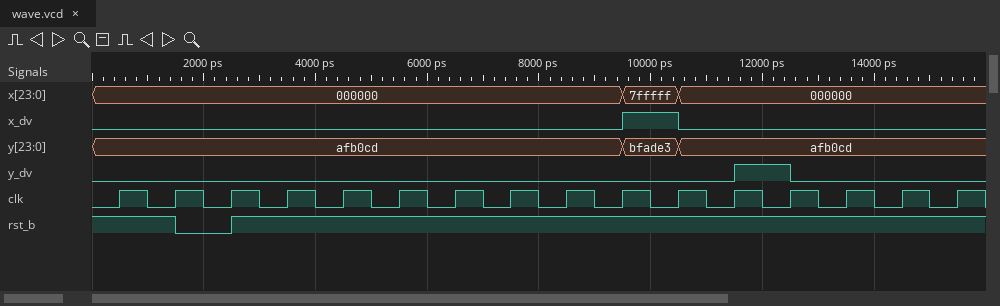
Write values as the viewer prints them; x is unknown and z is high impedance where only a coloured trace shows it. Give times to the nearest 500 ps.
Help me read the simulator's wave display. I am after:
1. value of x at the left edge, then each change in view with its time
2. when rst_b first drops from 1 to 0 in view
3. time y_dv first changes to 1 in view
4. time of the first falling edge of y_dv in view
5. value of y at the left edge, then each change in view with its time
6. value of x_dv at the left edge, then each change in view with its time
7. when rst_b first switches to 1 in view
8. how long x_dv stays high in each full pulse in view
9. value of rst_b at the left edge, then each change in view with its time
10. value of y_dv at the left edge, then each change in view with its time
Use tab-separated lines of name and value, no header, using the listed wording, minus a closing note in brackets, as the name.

value of x at the left edge, then each change in view with its time	000000, 7fffff at 9500 ps, 000000 at 10500 ps
when rst_b first drops from 1 to 0 in view	1500 ps
time y_dv first changes to 1 in view	11500 ps
time of the first falling edge of y_dv in view	12500 ps
value of y at the left edge, then each change in view with its time	afb0cd, bfade3 at 9500 ps, afb0cd at 10500 ps
value of x_dv at the left edge, then each change in view with its time	0, 1 at 9500 ps, 0 at 10500 ps
when rst_b first switches to 1 in view	2500 ps
how long x_dv stays high in each full pulse in view	1000 ps
value of rst_b at the left edge, then each change in view with its time	1, 0 at 1500 ps, 1 at 2500 ps
value of y_dv at the left edge, then each change in view with its time	0, 1 at 11500 ps, 0 at 12500 ps
